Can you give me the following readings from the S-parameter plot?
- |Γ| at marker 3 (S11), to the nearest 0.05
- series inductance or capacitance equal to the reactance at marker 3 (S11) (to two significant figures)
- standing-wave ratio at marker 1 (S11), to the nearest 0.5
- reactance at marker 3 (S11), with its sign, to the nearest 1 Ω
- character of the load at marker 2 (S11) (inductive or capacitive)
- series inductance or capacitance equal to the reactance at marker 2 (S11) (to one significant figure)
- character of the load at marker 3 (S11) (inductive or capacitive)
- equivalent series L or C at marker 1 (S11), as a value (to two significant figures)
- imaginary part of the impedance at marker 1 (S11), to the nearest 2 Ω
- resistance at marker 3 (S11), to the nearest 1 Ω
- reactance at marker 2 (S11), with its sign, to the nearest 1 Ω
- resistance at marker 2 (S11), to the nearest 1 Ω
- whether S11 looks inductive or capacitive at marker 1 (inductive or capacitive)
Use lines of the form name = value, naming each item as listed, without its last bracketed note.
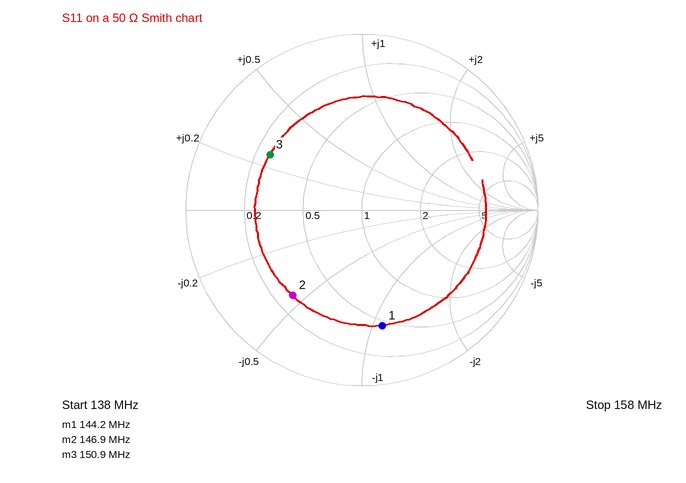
|Γ| at marker 3 (S11), to the nearest 0.05 = 0.60
series inductance or capacitance equal to the reactance at marker 3 (S11) = 14 nH
standing-wave ratio at marker 1 (S11), to the nearest 0.5 = 5.0
reactance at marker 3 (S11), with its sign, to the nearest 1 Ω = +13 Ω
character of the load at marker 2 (S11) = capacitive
series inductance or capacitance equal to the reactance at marker 2 (S11) = 50 pF
character of the load at marker 3 (S11) = inductive
equivalent series L or C at marker 1 (S11), as a value = 20 pF
imaginary part of the impedance at marker 1 (S11), to the nearest 2 Ω = -54 Ω
resistance at marker 3 (S11), to the nearest 1 Ω = 13 Ω
reactance at marker 2 (S11), with its sign, to the nearest 1 Ω = -22 Ω
resistance at marker 2 (S11), to the nearest 1 Ω = 14 Ω
whether S11 looks inductive or capacitive at marker 1 = capacitive
